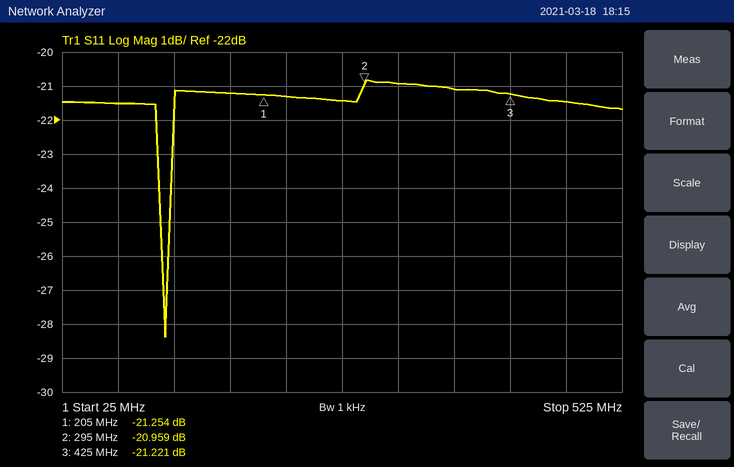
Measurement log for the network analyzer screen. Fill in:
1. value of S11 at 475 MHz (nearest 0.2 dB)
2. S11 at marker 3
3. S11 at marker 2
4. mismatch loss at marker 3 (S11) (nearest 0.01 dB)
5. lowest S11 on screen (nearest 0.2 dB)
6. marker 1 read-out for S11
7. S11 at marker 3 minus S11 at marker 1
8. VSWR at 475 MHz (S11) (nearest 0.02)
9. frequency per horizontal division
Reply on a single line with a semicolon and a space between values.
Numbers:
-21.4 dB; -21.221 dB; -20.959 dB; 0.03 dB; -28.4 dB; -21.254 dB; 0.033 dB; 1.18; 50 MHz
